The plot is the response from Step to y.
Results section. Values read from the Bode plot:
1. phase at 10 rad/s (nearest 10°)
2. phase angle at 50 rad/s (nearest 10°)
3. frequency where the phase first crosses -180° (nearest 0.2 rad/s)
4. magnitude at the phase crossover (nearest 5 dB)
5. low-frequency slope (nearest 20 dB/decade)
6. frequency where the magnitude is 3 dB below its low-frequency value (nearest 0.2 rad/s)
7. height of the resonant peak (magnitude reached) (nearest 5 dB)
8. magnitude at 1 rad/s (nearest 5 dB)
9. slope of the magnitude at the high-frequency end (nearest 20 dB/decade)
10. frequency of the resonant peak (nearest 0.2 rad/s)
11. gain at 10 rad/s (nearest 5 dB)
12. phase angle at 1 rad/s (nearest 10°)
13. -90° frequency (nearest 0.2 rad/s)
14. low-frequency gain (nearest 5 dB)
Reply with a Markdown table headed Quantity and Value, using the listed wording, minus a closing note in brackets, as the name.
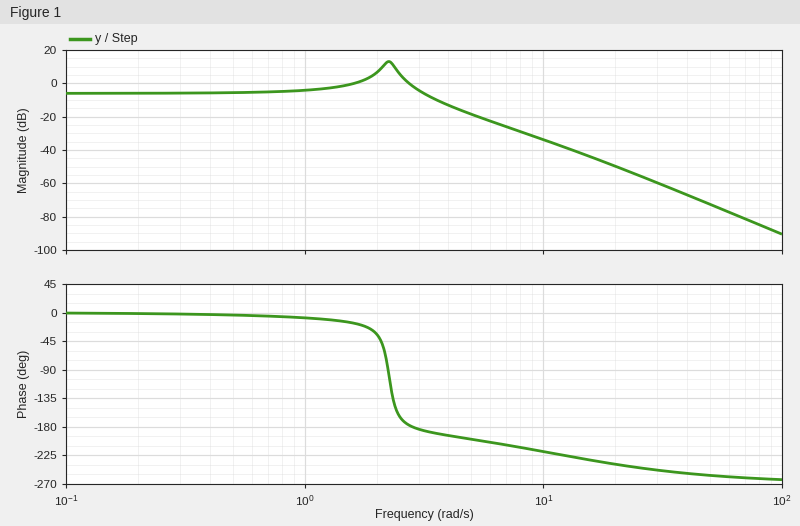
| Quantity | Value |
|---|---|
| phase at 10 rad/s | -220° |
| phase angle at 50 rad/s | -260° |
| frequency where the phase first crosses -180° | 2.8 rad/s |
| magnitude at the phase crossover | 0 dB |
| low-frequency slope | 0 dB/decade |
| frequency where the magnitude is 3 dB below its low-frequency value | 3.4 rad/s |
| height of the resonant peak (magnitude reached) | 15 dB |
| magnitude at 1 rad/s | -5 dB |
| slope of the magnitude at the high-frequency end | -60 dB/decade |
| frequency of the resonant peak | 2.2 rad/s |
| gain at 10 rad/s | -35 dB |
| phase angle at 1 rad/s | -10° |
| -90° frequency | 2.2 rad/s |
| low-frequency gain | -5 dB |
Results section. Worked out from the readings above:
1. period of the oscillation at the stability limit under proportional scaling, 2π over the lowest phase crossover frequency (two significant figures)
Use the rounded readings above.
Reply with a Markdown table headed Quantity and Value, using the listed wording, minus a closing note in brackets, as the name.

| Quantity | Value |
|---|---|
| period of the oscillation at the stability limit under proportional scaling, 2π over the lowest phase crossover frequency | 2.2 s |
